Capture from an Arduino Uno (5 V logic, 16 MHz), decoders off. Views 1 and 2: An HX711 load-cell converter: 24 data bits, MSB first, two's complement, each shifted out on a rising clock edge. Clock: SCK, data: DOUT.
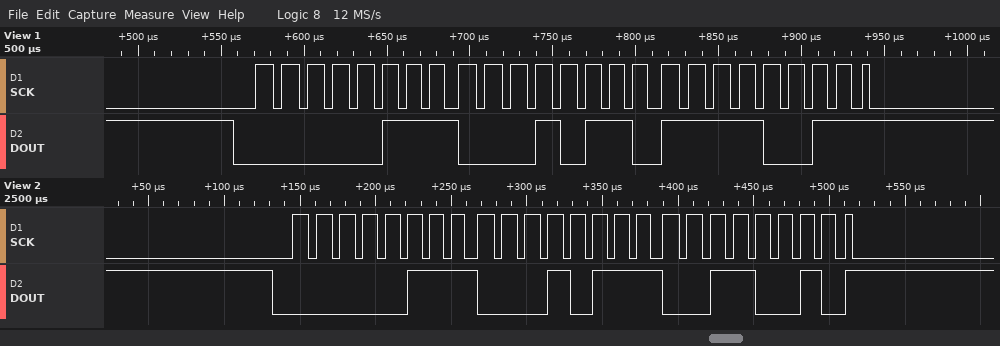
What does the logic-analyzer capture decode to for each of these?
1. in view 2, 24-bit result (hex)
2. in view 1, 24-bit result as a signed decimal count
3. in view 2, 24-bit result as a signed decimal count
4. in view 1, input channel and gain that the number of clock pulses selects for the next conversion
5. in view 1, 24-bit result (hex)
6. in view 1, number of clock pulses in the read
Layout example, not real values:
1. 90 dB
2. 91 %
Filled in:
1. 0x071732
2. 464627
3. 464690
4. channel A, gain 128
5. 0x0716F3
6. 25
